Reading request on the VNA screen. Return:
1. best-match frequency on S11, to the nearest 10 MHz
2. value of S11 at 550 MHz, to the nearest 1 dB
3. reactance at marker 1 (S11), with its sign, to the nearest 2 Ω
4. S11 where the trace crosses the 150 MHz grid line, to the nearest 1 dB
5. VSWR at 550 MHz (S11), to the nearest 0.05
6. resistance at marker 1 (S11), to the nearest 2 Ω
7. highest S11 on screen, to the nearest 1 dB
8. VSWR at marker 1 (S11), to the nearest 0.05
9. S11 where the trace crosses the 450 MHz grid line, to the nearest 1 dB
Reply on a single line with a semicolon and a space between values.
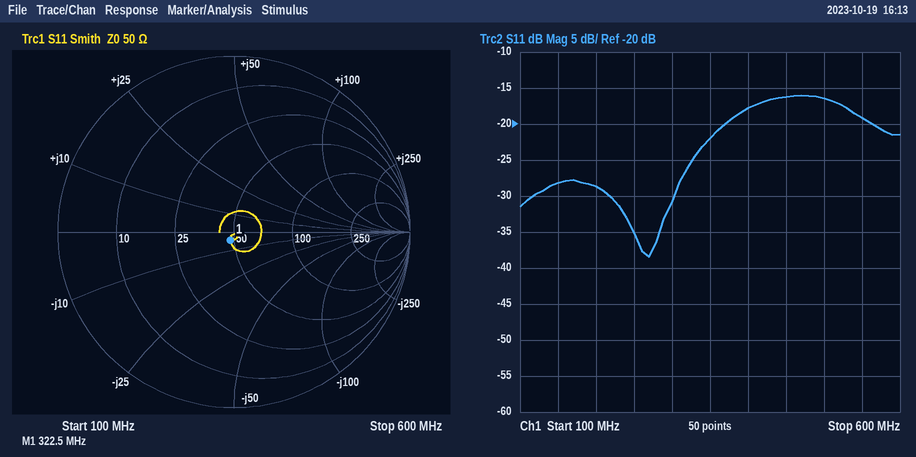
270 MHz; -19 dB; -4 Ω; -28 dB; 1.25; 48 Ω; -16 dB; 1.10; -16 dB
